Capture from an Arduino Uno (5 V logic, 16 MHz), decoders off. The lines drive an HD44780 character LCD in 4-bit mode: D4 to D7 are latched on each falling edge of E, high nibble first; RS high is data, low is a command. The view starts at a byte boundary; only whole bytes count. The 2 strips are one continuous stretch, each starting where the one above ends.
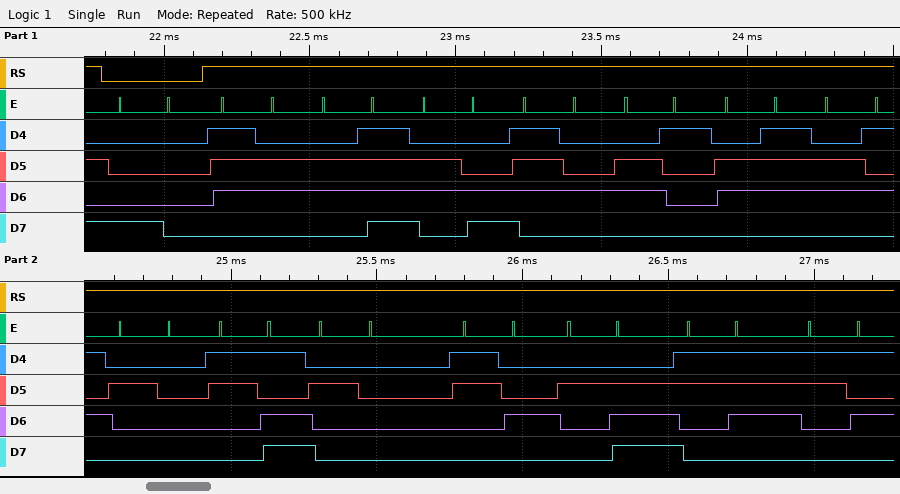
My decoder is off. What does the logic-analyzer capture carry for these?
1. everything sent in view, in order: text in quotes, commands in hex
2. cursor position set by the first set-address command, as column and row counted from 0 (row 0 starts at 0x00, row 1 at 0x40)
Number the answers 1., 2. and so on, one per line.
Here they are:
1. 0x80 "voltage = 4.75"
2. column 0, row 0
